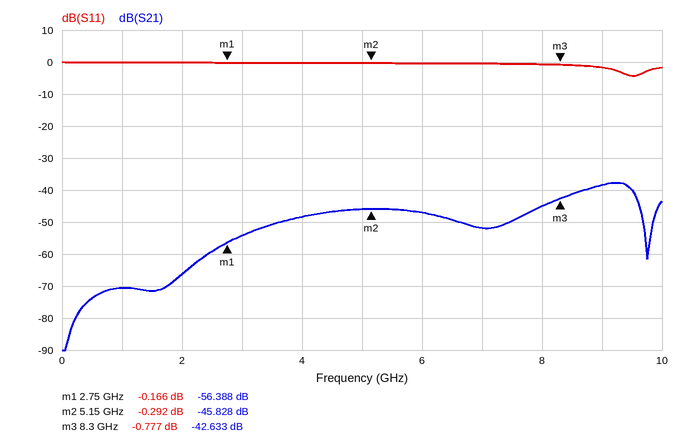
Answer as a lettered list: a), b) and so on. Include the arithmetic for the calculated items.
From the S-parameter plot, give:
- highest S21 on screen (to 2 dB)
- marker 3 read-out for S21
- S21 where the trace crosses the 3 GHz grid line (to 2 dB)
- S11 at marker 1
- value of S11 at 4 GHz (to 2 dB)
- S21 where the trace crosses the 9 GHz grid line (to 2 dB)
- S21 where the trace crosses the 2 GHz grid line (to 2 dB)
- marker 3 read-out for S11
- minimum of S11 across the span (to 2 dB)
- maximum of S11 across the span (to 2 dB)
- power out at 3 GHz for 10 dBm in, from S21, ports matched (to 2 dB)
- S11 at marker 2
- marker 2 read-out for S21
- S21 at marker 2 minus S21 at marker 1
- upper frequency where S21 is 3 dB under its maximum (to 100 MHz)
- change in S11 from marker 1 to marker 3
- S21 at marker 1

a) -38 dB
b) -42.633 dB
c) -54 dB
d) -0.166 dB
e) 0 dB
f) -38 dB
g) -66 dB
h) -0.777 dB
i) -4 dB
j) 0 dB
k) 10 dBm + (-54 dB) = -44 dBm
l) -0.292 dB
m) -45.828 dB
n) -45.828 − (-56.388) = 10.560 dB
o) 9.5 GHz
p) -0.777 − (-0.166) = -0.611 dB
q) -56.388 dB
